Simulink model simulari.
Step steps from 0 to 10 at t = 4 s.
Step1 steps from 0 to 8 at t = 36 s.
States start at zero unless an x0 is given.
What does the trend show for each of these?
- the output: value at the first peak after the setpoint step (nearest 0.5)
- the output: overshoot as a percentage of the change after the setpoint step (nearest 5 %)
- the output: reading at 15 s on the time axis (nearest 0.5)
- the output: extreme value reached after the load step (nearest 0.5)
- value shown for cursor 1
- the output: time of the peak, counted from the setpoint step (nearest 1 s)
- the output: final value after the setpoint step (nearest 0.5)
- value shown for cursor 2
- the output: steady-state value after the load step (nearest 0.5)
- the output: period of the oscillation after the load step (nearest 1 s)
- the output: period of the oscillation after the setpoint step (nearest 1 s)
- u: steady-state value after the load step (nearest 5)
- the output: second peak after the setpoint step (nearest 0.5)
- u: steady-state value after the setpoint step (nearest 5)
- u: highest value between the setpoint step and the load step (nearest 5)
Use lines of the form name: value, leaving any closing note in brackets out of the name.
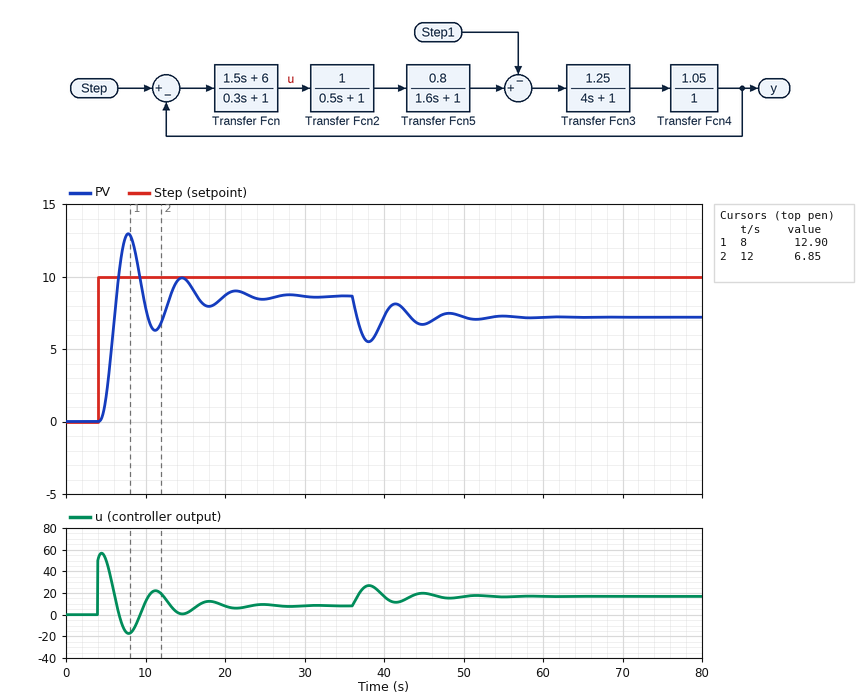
the output: value at the first peak after the setpoint step: 13.0
the output: overshoot as a percentage of the change after the setpoint step: 50 %
the output: reading at 15 s on the time axis: 10.0
the output: extreme value reached after the load step: 5.5
value shown for cursor 1: 12.90
the output: time of the peak, counted from the setpoint step: 4 s
the output: final value after the setpoint step: 8.5
value shown for cursor 2: 6.85
the output: steady-state value after the load step: 7.0
the output: period of the oscillation after the load step: 7 s
the output: period of the oscillation after the setpoint step: 7 s
u: steady-state value after the load step: 15
the output: second peak after the setpoint step: 10.0
u: steady-state value after the setpoint step: 10
u: highest value between the setpoint step and the load step: 55
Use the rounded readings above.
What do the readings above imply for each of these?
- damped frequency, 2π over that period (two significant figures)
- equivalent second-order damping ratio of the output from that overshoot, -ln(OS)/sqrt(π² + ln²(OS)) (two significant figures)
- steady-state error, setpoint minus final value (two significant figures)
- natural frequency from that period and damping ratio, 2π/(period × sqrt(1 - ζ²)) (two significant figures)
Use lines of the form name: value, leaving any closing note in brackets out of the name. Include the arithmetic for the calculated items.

damped frequency, 2π over that period: 2π / 7 = 0.90 rad/s
equivalent second-order damping ratio of the output from that overshoot, -ln(OS)/sqrt(π² + ln²(OS)): ln(0.5) = -0.693; 0.693 / sqrt(9.870 + 0.480) = 0.22
steady-state error, setpoint minus final value: 10 - 8.5 = 1.5
natural frequency from that period and damping ratio, 2π/(period × sqrt(1 - ζ²)): 2π / (7 × sqrt(1 - 0.22²)) = 0.92 rad/s
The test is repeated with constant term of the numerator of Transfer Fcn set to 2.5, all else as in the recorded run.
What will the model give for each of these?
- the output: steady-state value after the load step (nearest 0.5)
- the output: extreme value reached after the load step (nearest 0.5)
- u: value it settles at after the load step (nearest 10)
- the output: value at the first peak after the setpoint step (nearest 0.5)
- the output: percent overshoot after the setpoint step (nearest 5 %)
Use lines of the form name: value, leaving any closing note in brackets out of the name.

the output: steady-state value after the load step: 4.5
the output: extreme value reached after the load step: 3.5
u: value it settles at after the load step: 10
the output: value at the first peak after the setpoint step: 8.5
the output: percent overshoot after the setpoint step: 15 %
